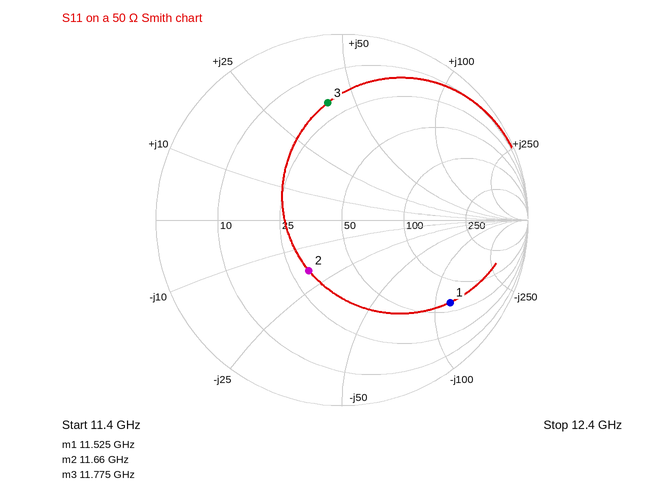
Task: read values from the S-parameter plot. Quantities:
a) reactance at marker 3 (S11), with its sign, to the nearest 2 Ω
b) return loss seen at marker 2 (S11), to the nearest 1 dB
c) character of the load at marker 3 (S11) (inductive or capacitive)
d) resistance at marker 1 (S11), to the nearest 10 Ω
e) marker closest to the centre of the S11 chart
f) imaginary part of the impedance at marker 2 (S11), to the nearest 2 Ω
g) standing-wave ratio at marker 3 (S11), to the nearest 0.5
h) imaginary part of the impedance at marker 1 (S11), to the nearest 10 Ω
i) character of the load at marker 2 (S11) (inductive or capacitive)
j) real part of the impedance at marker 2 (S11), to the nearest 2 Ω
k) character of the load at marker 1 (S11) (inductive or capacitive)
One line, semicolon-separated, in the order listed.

+40 Ω; 10 dB; inductive; 60 Ω; marker 2; -18 Ω; 4.5; -120 Ω; capacitive; 30 Ω; capacitive
